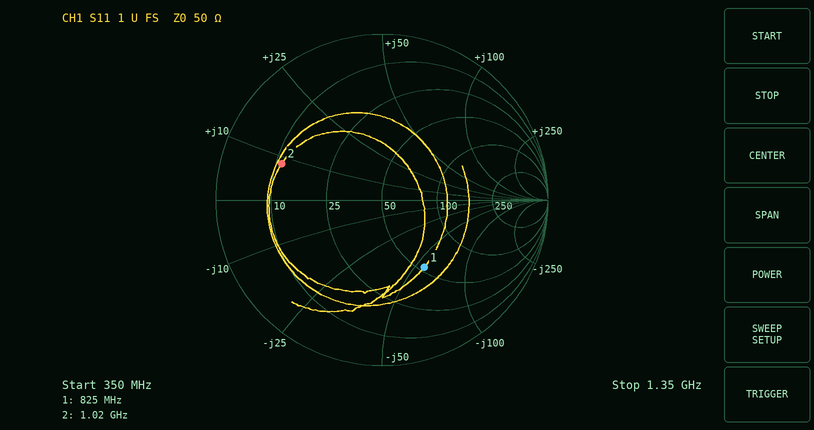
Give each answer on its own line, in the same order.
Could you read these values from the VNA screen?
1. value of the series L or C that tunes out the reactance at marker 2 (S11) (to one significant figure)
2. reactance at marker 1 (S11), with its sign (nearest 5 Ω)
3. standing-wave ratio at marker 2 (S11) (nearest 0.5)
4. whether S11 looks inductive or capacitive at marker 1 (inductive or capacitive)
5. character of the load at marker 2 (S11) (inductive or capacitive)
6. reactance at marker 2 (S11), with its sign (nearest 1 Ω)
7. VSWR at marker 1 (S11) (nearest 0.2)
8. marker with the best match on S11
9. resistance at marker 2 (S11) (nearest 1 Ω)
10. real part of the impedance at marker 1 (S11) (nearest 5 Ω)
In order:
20 pF
-55 Ω
4.5
capacitive
inductive
+8 Ω
2.8
marker 1
11 Ω
55 Ω
